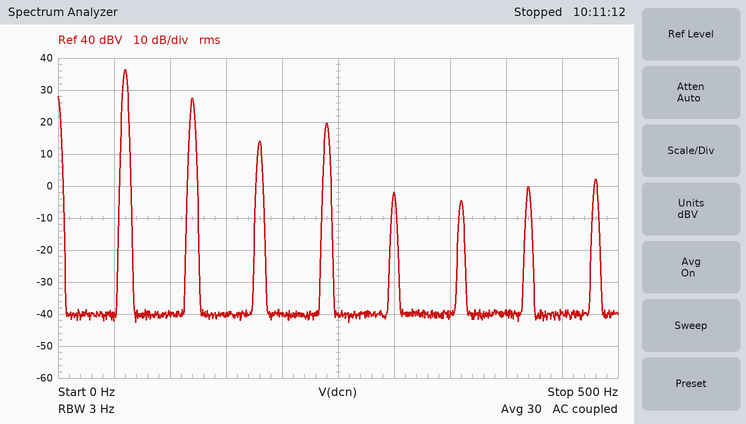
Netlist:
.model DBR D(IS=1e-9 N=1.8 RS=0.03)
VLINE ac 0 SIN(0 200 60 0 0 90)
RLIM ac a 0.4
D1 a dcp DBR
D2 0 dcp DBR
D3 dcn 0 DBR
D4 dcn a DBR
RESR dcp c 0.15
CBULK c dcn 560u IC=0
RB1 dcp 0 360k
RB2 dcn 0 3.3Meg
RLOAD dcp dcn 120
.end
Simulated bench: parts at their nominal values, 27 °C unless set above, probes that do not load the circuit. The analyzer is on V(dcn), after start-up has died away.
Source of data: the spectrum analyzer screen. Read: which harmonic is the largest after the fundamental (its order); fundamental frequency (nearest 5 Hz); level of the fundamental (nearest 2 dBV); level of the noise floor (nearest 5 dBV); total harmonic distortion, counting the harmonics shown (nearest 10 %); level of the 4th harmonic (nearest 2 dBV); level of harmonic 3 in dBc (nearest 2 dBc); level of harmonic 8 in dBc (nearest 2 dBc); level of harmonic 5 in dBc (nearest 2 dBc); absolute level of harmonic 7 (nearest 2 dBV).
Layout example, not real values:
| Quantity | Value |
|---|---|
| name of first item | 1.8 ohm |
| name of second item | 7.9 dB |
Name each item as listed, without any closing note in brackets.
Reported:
| Quantity | Value |
|---|---|
| which harmonic is the largest after the fundamental | 2 |
| fundamental frequency | 60 Hz |
| level of the fundamental | 36 dBV |
| level of the noise floor | -40 dBV |
| total harmonic distortion, counting the harmonics shown | 40 % |
| level of the 4th harmonic | 20 dBV |
| level of harmonic 3 in dBc | -22 dBc |
| level of harmonic 8 in dBc | -34 dBc |
| level of harmonic 5 in dBc | -38 dBc |
| absolute level of harmonic 7 | 0 dBV |
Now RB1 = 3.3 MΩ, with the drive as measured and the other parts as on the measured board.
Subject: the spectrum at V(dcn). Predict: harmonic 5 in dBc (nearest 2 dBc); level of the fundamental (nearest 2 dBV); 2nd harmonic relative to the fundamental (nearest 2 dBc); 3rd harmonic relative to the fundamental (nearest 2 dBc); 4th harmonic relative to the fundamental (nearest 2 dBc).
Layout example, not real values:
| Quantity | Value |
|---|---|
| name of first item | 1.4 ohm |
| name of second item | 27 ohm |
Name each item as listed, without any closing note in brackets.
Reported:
| Quantity | Value |
|---|---|
| harmonic 5 in dBc | -20 dBc |
| level of the fundamental | 36 dBV |
| 2nd harmonic relative to the fundamental | -28 dBc |
| 3rd harmonic relative to the fundamental | -10 dBc |
| 4th harmonic relative to the fundamental | -34 dBc |
